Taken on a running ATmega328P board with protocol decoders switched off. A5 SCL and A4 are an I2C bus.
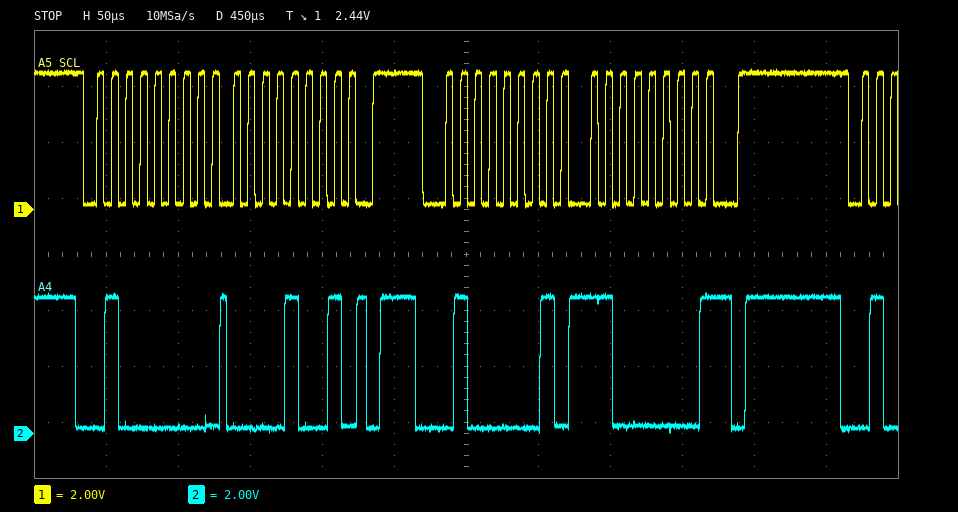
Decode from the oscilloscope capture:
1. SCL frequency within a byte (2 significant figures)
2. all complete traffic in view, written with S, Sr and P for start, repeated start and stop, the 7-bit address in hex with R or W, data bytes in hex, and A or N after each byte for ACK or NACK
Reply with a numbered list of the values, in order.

1. 100 kHz
2. S 20W A 09 A P S 20R A C0 N P
